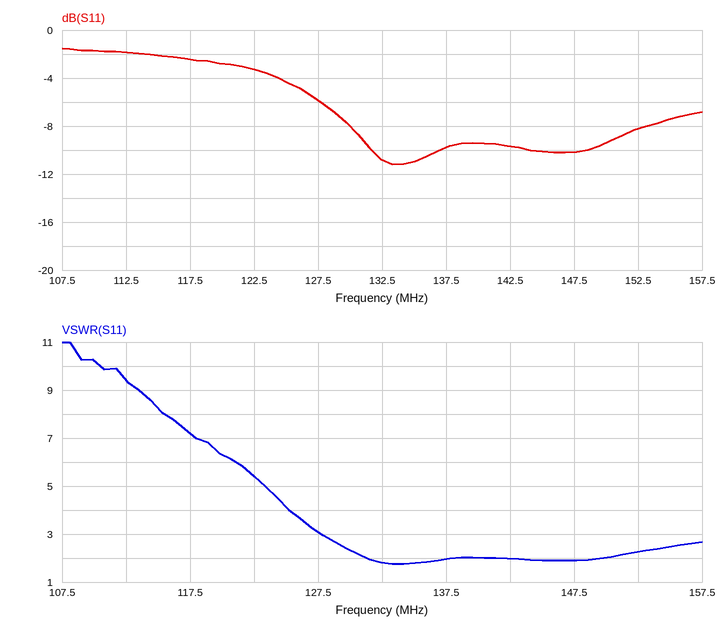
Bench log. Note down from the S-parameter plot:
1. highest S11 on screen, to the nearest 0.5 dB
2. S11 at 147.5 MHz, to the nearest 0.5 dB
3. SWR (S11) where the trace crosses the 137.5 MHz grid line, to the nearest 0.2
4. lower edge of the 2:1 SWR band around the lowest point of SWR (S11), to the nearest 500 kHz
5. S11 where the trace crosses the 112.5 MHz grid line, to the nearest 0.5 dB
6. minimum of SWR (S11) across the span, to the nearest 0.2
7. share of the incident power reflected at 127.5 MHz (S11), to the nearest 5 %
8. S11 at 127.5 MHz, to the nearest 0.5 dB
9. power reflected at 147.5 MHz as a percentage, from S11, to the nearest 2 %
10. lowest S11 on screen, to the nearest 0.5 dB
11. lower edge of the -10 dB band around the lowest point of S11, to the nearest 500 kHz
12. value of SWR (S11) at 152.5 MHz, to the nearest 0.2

-1.5 dB
-10.0 dB
2.0
131.5 MHz
-2.0 dB
1.8
25 %
-6.0 dB
10 %
-11.0 dB
131.5 MHz
2.2
